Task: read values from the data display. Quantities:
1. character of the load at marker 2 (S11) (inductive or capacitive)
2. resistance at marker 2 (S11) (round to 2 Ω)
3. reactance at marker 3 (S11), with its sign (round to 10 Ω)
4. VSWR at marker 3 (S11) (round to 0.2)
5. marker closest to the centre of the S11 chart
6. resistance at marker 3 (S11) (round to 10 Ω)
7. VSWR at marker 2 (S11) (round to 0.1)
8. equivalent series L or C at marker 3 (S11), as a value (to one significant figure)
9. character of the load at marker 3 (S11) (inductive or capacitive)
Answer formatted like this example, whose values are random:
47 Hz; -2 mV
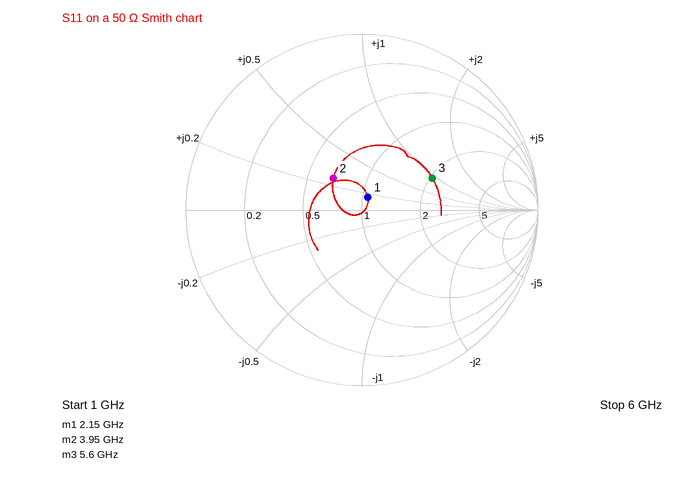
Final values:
inductive; 34 Ω; +50 Ω; 2.6; marker 1; 100 Ω; 1.6; 1 nH; inductive
